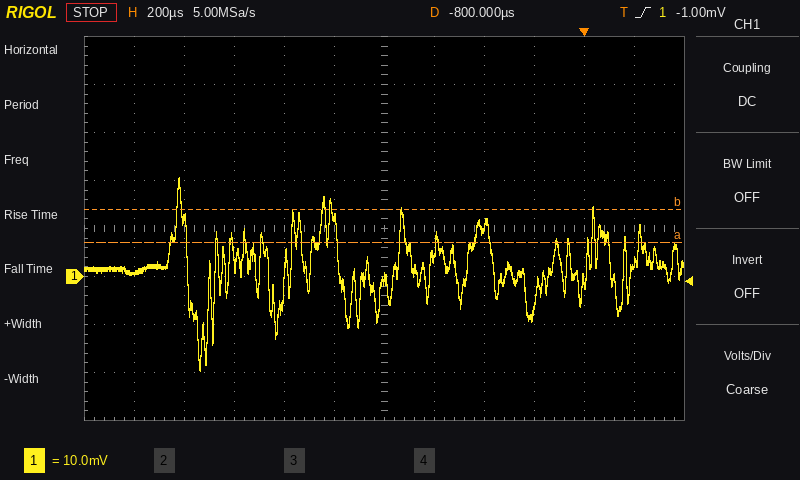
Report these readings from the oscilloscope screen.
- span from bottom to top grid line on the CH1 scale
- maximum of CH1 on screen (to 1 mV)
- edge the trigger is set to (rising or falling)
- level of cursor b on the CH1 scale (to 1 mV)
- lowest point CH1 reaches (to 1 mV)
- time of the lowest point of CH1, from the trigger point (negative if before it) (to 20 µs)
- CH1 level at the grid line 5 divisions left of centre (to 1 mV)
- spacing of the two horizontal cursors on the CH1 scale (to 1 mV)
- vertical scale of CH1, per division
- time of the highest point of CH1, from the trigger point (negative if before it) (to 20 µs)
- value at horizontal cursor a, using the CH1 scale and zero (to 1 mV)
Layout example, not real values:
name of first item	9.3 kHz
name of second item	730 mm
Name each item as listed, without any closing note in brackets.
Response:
span from bottom to top grid line on the CH1 scale	80 mV
maximum of CH1 on screen	21 mV
edge the trigger is set to	rising
level of cursor b on the CH1 scale	14 mV
lowest point CH1 reaches	-20 mV
time of the lowest point of CH1, from the trigger point (negative if before it)	-1.54 ms
CH1 level at the grid line 5 divisions left of centre	1 mV
spacing of the two horizontal cursors on the CH1 scale	7 mV
vertical scale of CH1, per division	10 mV
time of the highest point of CH1, from the trigger point (negative if before it)	-1.62 ms
value at horizontal cursor a, using the CH1 scale and zero	7 mV
